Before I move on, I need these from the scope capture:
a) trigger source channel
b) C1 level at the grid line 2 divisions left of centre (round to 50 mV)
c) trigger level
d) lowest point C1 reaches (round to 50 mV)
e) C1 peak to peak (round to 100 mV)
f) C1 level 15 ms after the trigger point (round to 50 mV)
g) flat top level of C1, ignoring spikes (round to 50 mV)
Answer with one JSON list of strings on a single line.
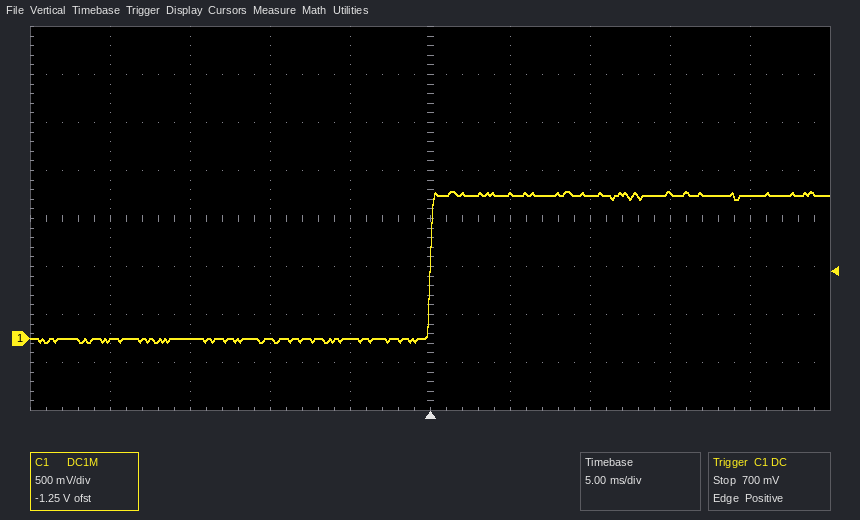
["C1", "0 mV", "700 mV", "-50 mV", "1.60 V", "1.50 V", "1.50 V"]
